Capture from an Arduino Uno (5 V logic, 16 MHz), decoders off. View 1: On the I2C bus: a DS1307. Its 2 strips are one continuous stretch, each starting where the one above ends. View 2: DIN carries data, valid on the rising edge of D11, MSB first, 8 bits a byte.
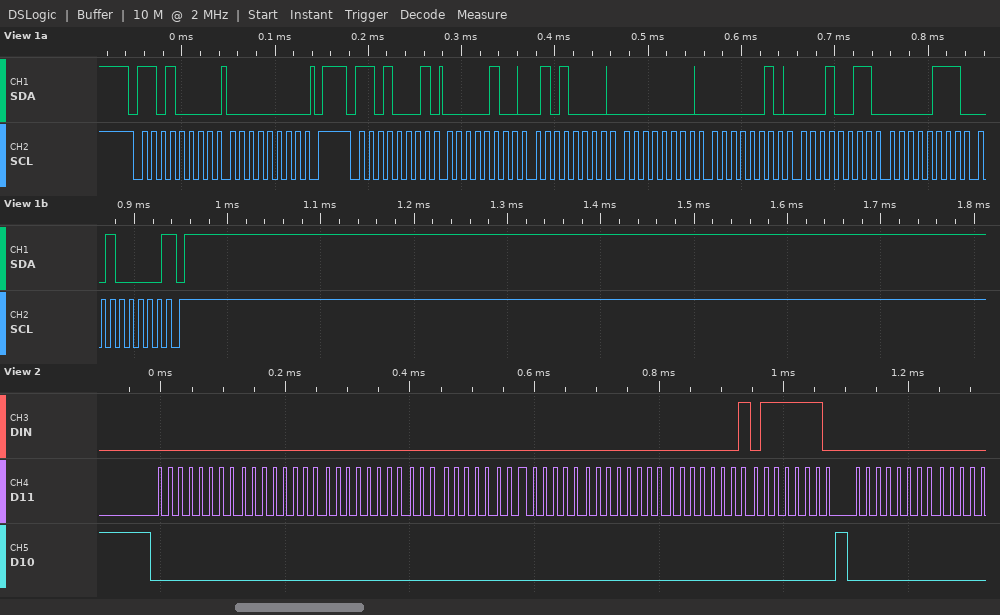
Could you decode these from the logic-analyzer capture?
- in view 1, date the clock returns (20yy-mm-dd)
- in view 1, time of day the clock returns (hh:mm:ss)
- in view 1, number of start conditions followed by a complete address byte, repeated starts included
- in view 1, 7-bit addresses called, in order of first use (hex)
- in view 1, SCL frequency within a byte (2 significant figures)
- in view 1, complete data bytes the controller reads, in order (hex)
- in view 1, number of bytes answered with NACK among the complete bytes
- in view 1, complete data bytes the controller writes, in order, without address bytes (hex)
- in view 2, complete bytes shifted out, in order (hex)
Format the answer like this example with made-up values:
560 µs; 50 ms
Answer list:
2020-07-13; 00:50:04; 2; 0x68; 100 kHz; 04 50 00 02 13 07 20; 1; 00; 00 00 00 00 00 00 01 7E 00
